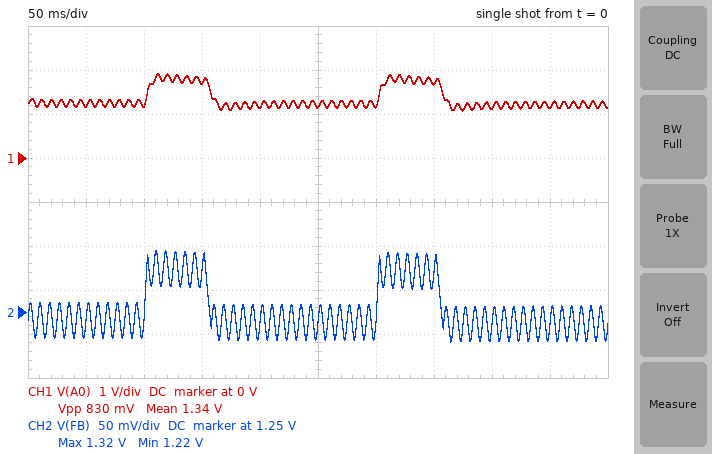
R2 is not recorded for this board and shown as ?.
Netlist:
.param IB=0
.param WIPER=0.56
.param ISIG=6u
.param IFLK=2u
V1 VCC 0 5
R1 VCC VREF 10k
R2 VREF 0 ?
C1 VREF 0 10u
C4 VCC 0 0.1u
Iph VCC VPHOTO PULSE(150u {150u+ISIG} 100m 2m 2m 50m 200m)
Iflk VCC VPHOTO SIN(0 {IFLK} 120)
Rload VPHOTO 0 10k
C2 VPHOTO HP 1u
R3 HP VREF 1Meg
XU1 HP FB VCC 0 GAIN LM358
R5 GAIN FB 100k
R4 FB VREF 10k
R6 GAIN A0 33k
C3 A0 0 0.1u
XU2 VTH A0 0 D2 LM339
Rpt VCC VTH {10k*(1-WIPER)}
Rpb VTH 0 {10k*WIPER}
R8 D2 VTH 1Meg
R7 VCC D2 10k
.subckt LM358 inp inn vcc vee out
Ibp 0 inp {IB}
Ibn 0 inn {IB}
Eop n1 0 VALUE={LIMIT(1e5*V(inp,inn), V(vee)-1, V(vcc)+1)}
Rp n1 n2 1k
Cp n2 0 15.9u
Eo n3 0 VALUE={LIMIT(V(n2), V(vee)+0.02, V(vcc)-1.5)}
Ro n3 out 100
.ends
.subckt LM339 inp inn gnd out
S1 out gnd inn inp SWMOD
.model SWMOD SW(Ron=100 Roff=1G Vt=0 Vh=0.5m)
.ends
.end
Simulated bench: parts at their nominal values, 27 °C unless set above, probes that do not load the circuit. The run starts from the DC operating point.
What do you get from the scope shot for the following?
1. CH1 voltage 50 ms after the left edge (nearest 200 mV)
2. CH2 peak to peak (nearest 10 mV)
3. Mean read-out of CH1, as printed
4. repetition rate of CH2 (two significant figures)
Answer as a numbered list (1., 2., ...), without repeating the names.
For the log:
1. 1.2 V
2. 100 mV
3. 1.34 V
4. 5.0 Hz
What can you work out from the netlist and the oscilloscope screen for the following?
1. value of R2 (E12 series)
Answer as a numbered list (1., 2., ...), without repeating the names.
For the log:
1. 3.3 kΩ
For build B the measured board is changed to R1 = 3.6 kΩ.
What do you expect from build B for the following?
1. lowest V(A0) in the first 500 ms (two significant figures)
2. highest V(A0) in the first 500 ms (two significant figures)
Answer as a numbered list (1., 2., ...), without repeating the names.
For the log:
1. 2.2 V
2. 3.1 V
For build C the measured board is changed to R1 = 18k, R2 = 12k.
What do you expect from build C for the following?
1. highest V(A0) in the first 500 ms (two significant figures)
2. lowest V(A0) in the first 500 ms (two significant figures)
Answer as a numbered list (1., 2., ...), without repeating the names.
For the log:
1. 2.7 V
2. 1.8 V
